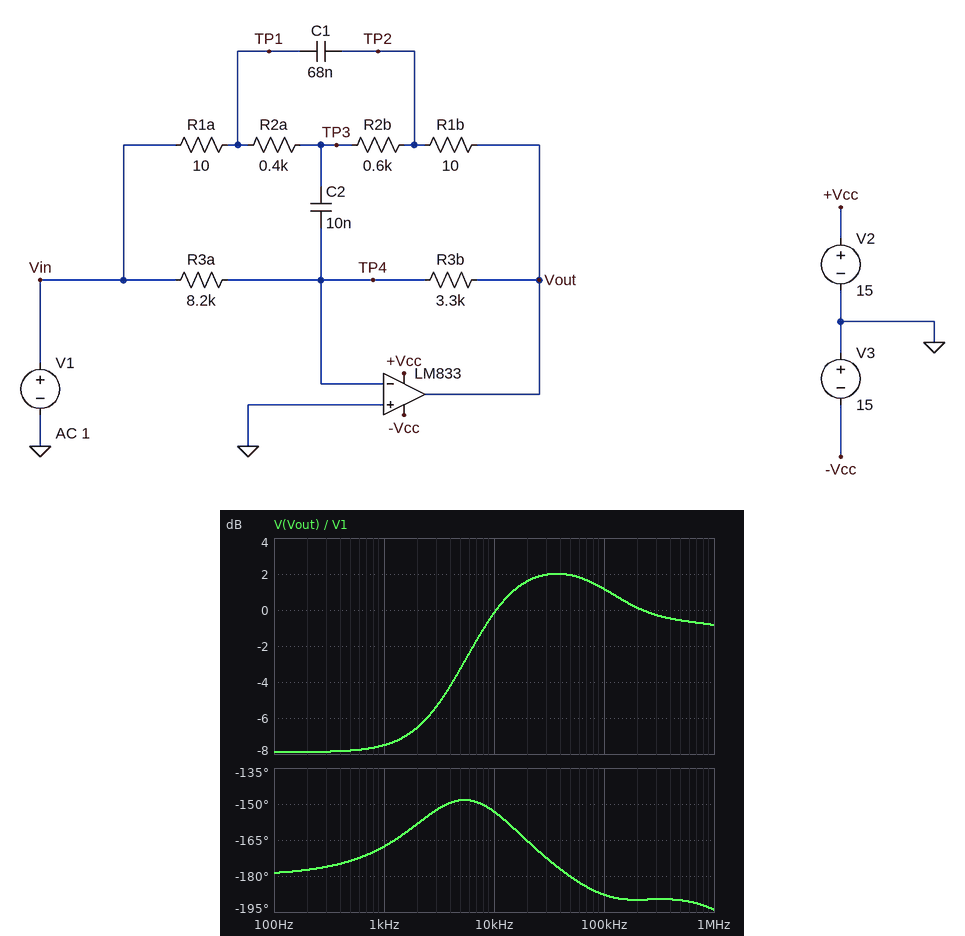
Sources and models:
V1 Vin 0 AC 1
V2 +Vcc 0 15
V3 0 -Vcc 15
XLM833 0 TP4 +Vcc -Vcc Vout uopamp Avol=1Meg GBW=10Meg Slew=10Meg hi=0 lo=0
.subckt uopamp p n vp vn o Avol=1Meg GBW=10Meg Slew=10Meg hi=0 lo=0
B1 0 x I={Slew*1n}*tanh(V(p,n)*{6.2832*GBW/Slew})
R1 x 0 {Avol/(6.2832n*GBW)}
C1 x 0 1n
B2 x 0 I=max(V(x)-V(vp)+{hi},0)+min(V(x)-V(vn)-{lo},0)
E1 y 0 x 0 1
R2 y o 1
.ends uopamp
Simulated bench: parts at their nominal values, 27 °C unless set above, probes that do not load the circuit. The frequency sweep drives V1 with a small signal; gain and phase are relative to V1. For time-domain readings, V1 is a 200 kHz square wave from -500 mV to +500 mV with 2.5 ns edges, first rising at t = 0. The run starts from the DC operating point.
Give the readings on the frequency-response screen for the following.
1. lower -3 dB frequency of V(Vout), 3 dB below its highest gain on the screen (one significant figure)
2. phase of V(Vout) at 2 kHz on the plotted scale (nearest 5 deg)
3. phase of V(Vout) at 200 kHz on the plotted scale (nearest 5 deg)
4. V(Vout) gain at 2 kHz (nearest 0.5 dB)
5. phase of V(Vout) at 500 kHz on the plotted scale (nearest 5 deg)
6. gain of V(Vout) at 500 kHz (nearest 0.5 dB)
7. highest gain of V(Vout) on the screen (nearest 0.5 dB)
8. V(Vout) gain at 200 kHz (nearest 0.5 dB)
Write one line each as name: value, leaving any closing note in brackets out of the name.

lower -3 dB frequency of V(Vout), 3 dB below its highest gain on the screen: 8 kHz
phase of V(Vout) at 2 kHz on the plotted scale: -160 deg
phase of V(Vout) at 200 kHz on the plotted scale: -190 deg
V(Vout) gain at 2 kHz: -6.5 dB
phase of V(Vout) at 500 kHz on the plotted scale: -190 deg
gain of V(Vout) at 500 kHz: -0.5 dB
highest gain of V(Vout) on the screen: 2.0 dB
V(Vout) gain at 200 kHz: 0 dB
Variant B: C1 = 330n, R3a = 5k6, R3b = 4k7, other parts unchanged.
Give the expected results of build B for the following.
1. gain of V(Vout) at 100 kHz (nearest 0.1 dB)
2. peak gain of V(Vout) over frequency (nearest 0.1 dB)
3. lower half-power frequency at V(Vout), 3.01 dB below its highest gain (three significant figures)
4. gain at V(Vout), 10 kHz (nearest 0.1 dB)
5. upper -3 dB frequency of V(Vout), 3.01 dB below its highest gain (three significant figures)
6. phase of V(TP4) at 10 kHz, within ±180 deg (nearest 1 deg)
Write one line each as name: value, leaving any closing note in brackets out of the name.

gain of V(Vout) at 100 kHz: 0.1 dB
peak gain of V(Vout) over frequency: 2.2 dB
lower half-power frequency at V(Vout), 3.01 dB below its highest gain: 2.19 kHz
gain at V(Vout), 10 kHz: 2.0 dB
upper -3 dB frequency of V(Vout), 3.01 dB below its highest gain: 2.02 MHz
phase of V(TP4) at 10 kHz, within ±180 deg: 98 deg
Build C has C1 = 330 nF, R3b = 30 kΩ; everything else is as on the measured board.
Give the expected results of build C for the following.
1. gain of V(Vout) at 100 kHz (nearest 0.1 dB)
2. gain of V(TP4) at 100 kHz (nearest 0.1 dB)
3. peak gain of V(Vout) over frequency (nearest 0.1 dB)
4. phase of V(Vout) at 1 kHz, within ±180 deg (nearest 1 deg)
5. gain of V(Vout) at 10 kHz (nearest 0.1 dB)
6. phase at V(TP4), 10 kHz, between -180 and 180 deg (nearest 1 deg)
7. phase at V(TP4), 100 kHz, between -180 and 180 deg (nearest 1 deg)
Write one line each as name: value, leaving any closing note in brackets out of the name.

gain of V(Vout) at 100 kHz: 0.6 dB
gain of V(TP4) at 100 kHz: -38.7 dB
peak gain of V(Vout) over frequency: 11.3 dB
phase of V(Vout) at 1 kHz, within ±180 deg: 160 deg
gain of V(Vout) at 10 kHz: 3.8 dB
phase at V(TP4), 10 kHz, between -180 and 180 deg: 74 deg
phase at V(TP4), 100 kHz, between -180 and 180 deg: 84 deg
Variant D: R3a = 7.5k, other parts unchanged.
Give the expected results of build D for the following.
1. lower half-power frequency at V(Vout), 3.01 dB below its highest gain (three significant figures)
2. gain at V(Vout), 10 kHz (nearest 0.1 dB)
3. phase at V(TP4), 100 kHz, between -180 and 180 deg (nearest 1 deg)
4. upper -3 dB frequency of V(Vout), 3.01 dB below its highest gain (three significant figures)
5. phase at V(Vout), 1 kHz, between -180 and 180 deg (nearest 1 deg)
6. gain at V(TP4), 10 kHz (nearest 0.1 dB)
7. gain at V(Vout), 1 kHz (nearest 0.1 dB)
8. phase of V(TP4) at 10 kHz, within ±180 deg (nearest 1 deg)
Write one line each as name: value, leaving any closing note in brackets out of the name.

lower half-power frequency at V(Vout), 3.01 dB below its highest gain: 7.94 kHz
gain at V(Vout), 10 kHz: -0.1 dB
phase at V(TP4), 100 kHz, between -180 and 180 deg: 85 deg
upper -3 dB frequency of V(Vout), 3.01 dB below its highest gain: 1.35 MHz
phase at V(Vout), 1 kHz, between -180 and 180 deg: -169 deg
gain at V(TP4), 10 kHz: -60.0 dB
gain at V(Vout), 1 kHz: -6.8 dB
phase of V(TP4) at 10 kHz, within ±180 deg: 116 deg
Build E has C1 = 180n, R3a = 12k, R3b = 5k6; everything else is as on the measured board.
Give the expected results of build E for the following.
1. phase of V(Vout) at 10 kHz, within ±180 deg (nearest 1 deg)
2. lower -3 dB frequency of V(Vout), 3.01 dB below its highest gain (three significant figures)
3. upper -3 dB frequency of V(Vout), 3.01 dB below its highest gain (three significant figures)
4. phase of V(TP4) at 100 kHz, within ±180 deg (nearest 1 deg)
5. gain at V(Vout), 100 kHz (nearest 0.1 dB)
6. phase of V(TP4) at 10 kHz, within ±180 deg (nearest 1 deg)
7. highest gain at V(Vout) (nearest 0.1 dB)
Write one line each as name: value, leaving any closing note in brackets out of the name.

phase of V(Vout) at 10 kHz, within ±180 deg: -164 deg
lower -3 dB frequency of V(Vout), 3.01 dB below its highest gain: 4.65 kHz
upper -3 dB frequency of V(Vout), 3.01 dB below its highest gain: 1.52 MHz
phase of V(TP4) at 100 kHz, within ±180 deg: 85 deg
gain at V(Vout), 100 kHz: 0.2 dB
phase of V(TP4) at 10 kHz, within ±180 deg: 107 deg
highest gain at V(Vout): 2.2 dB
